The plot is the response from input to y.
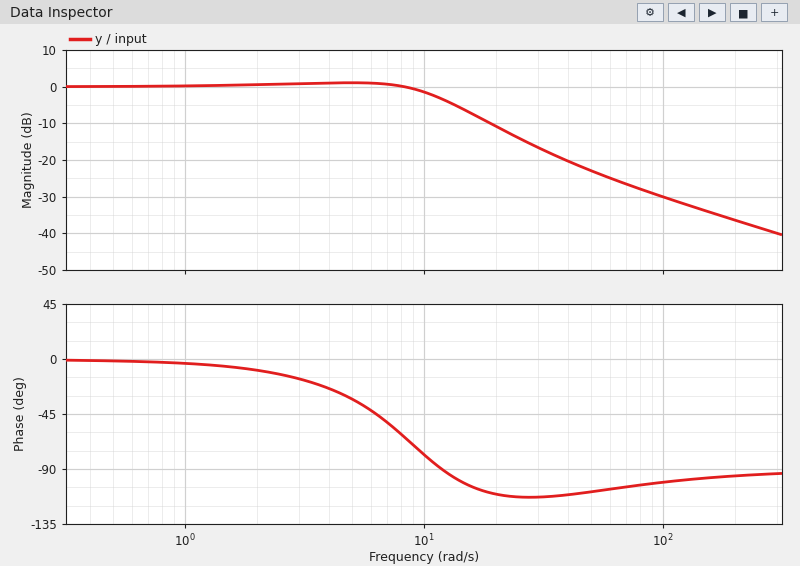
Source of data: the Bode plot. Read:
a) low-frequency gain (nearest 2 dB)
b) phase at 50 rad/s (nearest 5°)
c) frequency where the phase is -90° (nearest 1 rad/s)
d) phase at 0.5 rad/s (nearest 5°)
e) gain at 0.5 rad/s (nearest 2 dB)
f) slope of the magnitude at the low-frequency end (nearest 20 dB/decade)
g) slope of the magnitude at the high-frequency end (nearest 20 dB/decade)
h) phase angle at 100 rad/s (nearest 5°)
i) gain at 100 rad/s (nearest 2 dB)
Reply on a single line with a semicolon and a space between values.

0 dB; -110°; 12 rad/s; 0°; 0 dB; 0 dB/decade; -20 dB/decade; -100°; -30 dB
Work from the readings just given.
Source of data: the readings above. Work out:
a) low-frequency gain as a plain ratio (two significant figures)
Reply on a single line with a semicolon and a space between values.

1.0
